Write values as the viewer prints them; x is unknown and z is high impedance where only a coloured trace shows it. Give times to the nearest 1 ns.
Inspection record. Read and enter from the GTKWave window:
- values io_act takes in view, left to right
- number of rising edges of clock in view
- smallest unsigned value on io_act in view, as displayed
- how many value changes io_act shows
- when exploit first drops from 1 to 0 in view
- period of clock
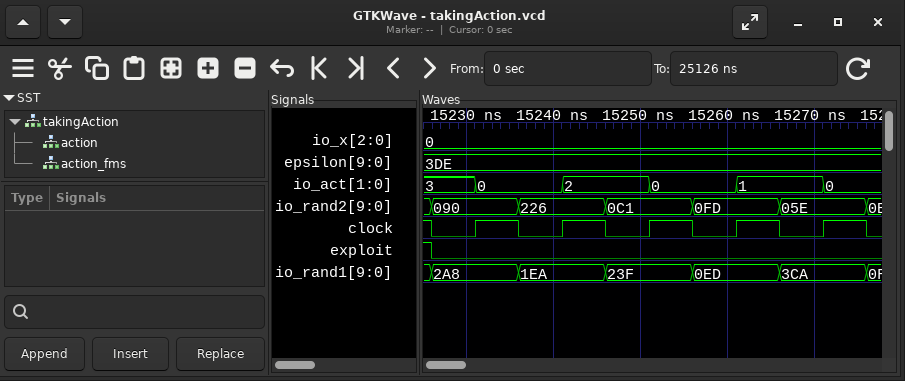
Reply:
3, 0, 2, 0, 1, 0
5
0
5
15226 ns
10 ns
